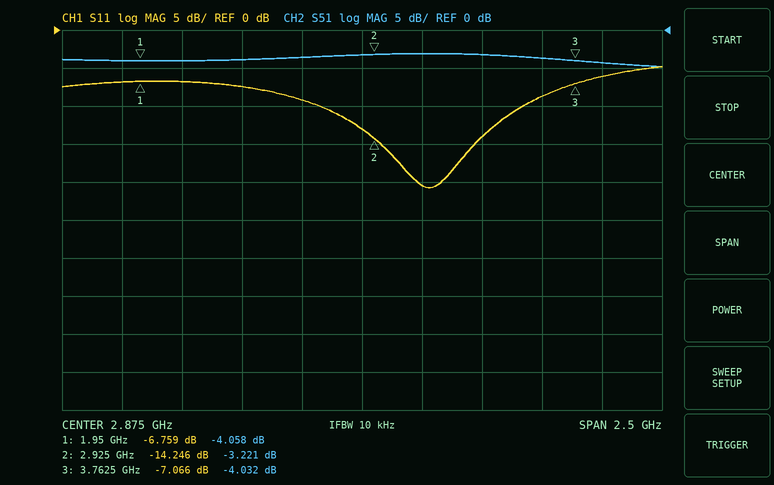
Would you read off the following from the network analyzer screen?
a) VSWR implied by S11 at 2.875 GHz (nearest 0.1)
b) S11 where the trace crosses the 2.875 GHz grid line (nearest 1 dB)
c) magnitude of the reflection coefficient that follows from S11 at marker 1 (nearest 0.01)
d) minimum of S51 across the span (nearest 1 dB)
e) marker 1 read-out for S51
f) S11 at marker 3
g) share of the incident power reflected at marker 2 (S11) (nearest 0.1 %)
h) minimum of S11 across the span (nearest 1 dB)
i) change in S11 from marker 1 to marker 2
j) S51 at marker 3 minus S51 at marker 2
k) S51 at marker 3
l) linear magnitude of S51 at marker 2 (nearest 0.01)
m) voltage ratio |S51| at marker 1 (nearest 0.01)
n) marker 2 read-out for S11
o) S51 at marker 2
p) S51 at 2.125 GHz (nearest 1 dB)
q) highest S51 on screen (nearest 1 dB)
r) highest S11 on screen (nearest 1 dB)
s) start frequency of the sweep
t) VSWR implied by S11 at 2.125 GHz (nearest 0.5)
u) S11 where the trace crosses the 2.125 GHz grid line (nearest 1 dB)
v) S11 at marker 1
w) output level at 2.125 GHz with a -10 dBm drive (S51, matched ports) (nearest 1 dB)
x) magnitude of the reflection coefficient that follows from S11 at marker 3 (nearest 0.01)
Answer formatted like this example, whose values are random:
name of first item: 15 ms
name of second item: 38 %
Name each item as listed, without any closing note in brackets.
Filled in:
VSWR implied by S11 at 2.875 GHz: 1.6
S11 where the trace crosses the 2.875 GHz grid line: -13 dB
magnitude of the reflection coefficient that follows from S11 at marker 1: 0.46
minimum of S51 across the span: -5 dB
marker 1 read-out for S51: -4.058 dB
S11 at marker 3: -7.066 dB
share of the incident power reflected at marker 2 (S11): 3.8 %
minimum of S11 across the span: -21 dB
change in S11 from marker 1 to marker 2: -7.487 dB
S51 at marker 3 minus S51 at marker 2: -0.811 dB
S51 at marker 3: -4.032 dB
linear magnitude of S51 at marker 2: 0.69
voltage ratio |S51| at marker 1: 0.63
marker 2 read-out for S11: -14.246 dB
S51 at marker 2: -3.221 dB
S51 at 2.125 GHz: -4 dB
highest S51 on screen: -3 dB
highest S11 on screen: -5 dB
start frequency of the sweep: 1.625 GHz
VSWR implied by S11 at 2.125 GHz: 2.5
S11 where the trace crosses the 2.125 GHz grid line: -7 dB
S11 at marker 1: -6.759 dB
output level at 2.125 GHz with a -10 dBm drive (S51, matched ports): -14 dBm
magnitude of the reflection coefficient that follows from S11 at marker 3: 0.44
